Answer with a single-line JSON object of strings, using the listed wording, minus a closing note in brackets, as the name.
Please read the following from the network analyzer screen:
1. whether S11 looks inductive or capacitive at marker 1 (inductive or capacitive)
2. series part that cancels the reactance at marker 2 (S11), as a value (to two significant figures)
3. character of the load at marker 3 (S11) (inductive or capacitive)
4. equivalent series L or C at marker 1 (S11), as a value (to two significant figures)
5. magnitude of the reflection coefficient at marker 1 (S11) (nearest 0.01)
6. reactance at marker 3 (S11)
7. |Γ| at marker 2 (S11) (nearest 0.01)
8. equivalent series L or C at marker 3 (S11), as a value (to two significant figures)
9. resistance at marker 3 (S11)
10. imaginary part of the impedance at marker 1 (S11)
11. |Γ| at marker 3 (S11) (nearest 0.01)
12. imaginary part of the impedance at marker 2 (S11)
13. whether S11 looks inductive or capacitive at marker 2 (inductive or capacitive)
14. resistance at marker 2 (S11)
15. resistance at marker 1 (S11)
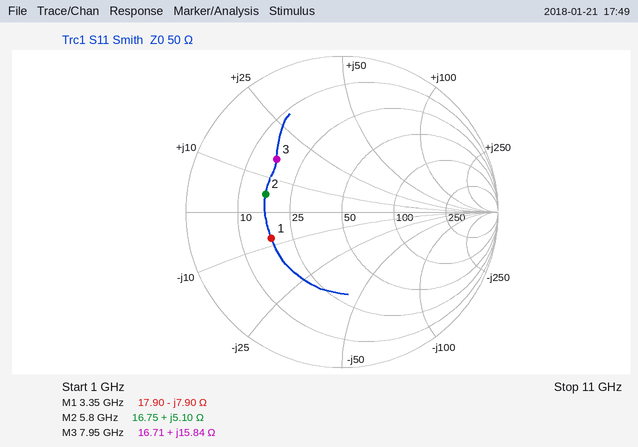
{"whether S11 looks inductive or capacitive at marker 1": "capacitive", "series part that cancels the reactance at marker 2 (S11), as a value": "5.4 pF", "character of the load at marker 3 (S11)": "inductive", "equivalent series L or C at marker 1 (S11), as a value": "6.0 pF", "magnitude of the reflection coefficient at marker 1 (S11)": "0.48", "reactance at marker 3": "+15.84 Ω", "|Γ| at marker 2 (S11)": "0.50", "equivalent series L or C at marker 3 (S11), as a value": "320 pH", "resistance at marker 3": "16.71 Ω", "imaginary part of the impedance at marker 1": "-7.90 Ω", "|Γ| at marker 3 (S11)": "0.54", "imaginary part of the impedance at marker 2": "+5.10 Ω", "whether S11 looks inductive or capacitive at marker 2": "inductive", "resistance at marker 2": "16.75 Ω", "resistance at marker 1": "17.90 Ω"}
